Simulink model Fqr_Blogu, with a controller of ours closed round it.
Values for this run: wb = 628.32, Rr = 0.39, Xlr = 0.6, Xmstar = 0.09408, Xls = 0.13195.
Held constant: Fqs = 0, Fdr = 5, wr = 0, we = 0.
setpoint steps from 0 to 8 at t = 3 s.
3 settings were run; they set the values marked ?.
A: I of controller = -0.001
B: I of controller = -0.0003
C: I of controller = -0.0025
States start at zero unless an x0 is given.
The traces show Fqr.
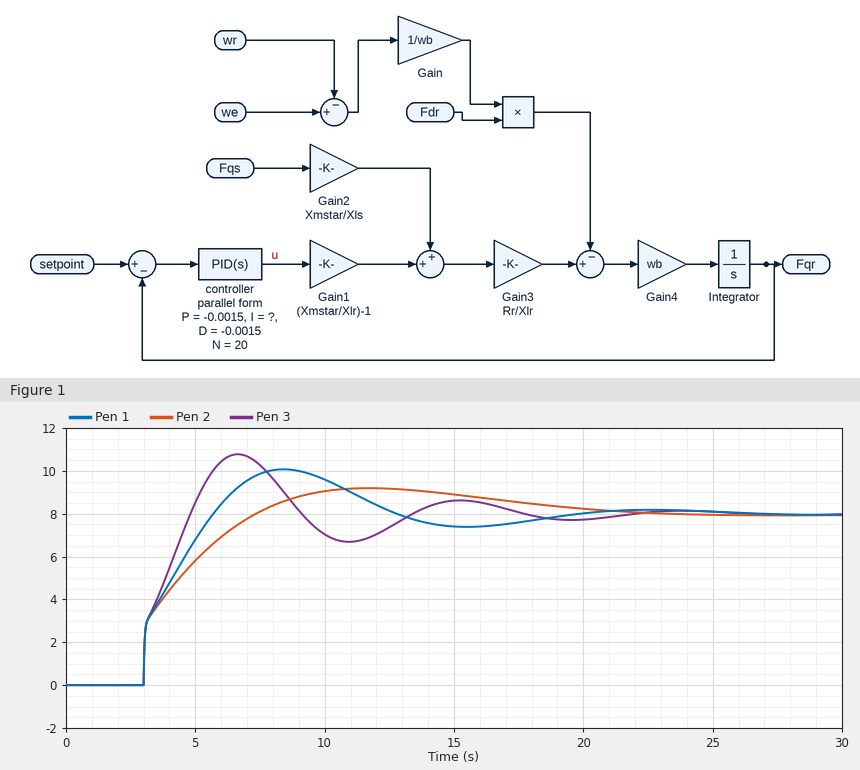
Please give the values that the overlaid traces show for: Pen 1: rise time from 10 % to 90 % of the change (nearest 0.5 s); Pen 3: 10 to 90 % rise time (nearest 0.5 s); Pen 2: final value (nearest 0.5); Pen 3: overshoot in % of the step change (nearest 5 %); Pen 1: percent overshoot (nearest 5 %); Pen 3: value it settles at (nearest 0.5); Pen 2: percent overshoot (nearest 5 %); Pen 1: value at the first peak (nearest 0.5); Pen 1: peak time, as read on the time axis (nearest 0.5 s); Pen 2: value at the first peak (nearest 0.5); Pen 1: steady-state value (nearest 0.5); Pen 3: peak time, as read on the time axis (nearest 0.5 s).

2.0 s
1.5 s
8.0
35 %
25 %
8.0
15 %
10.0
8.5 s
9.0
8.0
6.5 s
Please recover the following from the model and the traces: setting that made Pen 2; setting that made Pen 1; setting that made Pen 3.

B
A
C
